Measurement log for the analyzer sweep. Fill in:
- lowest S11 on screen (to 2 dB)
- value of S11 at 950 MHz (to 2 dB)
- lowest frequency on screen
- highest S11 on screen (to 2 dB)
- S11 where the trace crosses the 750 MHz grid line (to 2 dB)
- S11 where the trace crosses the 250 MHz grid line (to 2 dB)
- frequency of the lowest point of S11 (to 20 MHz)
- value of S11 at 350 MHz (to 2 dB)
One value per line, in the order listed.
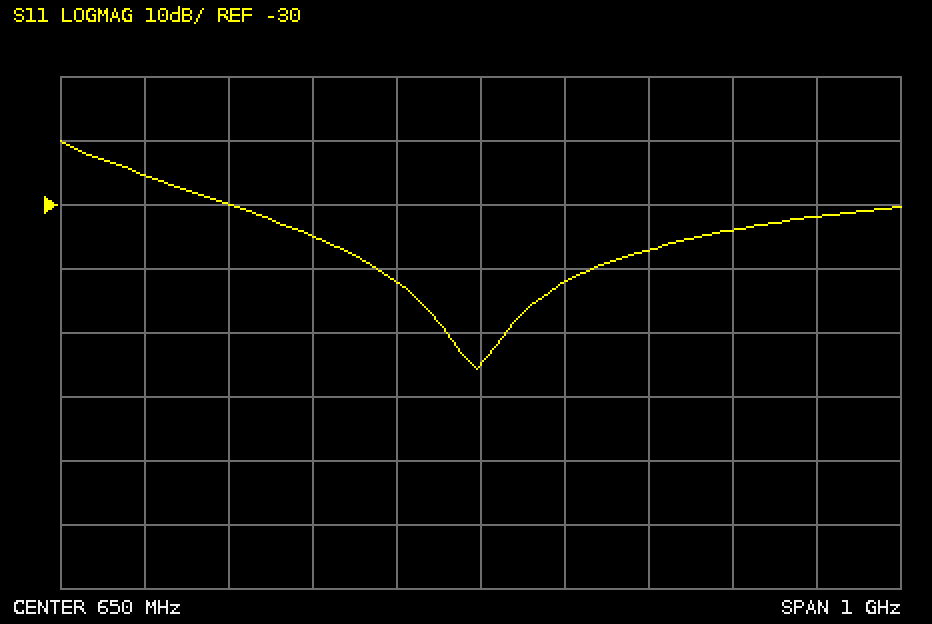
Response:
-56 dB
-34 dB
150 MHz
-20 dB
-42 dB
-26 dB
640 MHz
-30 dB
